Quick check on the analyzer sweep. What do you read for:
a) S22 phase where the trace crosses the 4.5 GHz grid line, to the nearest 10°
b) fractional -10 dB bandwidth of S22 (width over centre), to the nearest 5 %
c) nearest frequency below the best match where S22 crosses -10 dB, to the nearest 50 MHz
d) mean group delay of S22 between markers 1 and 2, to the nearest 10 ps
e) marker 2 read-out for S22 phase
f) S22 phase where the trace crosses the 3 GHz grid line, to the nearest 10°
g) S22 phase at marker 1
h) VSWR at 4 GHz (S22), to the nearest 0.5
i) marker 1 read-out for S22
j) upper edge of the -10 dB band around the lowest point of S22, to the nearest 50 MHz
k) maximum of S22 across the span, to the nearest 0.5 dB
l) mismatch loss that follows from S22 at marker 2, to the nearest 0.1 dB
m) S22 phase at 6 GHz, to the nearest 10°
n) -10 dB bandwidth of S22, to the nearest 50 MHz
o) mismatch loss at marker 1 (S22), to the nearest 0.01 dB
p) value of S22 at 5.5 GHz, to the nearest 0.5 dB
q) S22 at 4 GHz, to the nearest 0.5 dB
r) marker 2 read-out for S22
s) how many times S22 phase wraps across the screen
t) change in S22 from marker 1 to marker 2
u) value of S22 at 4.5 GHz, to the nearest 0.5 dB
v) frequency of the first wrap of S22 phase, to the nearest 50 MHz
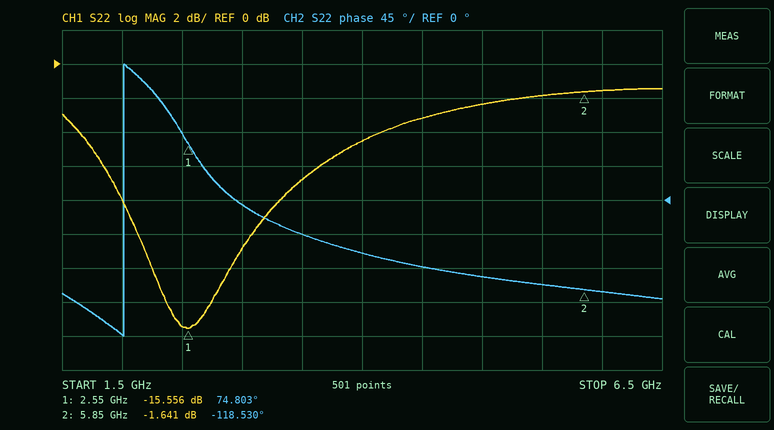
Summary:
-90°
35 %
2.15 GHz
160 ps
-118.530°
-10°
74.803°
4.0
-15.556 dB
3.10 GHz
-1.5 dB
5.0 dB
-120°
950 MHz
0.12 dB
-2.0 dB
-4.5 dB
-1.641 dB
1
13.915 dB
-3.0 dB
2.00 GHz
